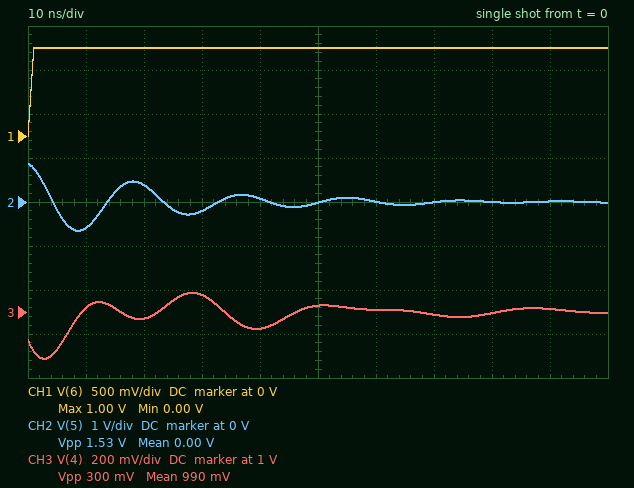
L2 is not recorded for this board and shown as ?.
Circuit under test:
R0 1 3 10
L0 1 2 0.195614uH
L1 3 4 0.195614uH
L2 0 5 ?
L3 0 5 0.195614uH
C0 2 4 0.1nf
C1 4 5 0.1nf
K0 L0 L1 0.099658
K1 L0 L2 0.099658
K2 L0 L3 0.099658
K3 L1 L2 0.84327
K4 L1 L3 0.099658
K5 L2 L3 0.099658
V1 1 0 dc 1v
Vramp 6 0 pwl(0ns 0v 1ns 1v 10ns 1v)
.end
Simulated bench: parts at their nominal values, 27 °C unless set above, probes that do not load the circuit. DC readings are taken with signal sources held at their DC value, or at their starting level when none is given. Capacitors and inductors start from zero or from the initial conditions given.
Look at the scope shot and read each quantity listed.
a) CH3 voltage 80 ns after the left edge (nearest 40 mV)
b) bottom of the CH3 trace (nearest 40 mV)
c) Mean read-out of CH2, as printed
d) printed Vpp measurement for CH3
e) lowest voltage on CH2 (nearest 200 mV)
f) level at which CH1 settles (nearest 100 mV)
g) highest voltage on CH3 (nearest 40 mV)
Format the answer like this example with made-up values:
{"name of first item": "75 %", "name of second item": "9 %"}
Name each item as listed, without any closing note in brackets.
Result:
{"CH3 voltage 80 ns after the left edge": "1.00 V", "bottom of the CH3 trace": "800 mV", "Mean read-out of CH2, as printed": "0.00 V", "printed Vpp measurement for CH3": "300 mV", "lowest voltage on CH2": "-600 mV", "level at which CH1 settles": "1.0 V", "highest voltage on CH3": "1.08 V"}
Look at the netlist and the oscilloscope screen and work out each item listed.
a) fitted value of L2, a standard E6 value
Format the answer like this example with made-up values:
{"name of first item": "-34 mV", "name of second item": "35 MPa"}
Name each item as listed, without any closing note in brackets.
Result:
{"fitted value of L2, a standard E6 value": "470 nH"}
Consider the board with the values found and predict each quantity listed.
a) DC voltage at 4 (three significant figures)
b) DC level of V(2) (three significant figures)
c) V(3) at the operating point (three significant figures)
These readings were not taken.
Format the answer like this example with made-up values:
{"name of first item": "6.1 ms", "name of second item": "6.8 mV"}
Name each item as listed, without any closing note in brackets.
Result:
{"DC voltage at 4": "1.00 V", "DC level of V(2)": "1.00 V", "V(3) at the operating point": "1.00 V"}
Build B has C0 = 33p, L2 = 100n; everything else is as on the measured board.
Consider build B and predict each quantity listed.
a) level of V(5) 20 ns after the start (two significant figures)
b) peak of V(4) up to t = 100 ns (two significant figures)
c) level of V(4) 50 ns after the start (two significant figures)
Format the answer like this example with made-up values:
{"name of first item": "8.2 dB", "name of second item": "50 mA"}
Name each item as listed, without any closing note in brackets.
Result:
{"level of V(5) 20 ns after the start": "-160 mV", "peak of V(4) up to t = 100 ns": "1.4 V", "level of V(4) 50 ns after the start": "920 mV"}
